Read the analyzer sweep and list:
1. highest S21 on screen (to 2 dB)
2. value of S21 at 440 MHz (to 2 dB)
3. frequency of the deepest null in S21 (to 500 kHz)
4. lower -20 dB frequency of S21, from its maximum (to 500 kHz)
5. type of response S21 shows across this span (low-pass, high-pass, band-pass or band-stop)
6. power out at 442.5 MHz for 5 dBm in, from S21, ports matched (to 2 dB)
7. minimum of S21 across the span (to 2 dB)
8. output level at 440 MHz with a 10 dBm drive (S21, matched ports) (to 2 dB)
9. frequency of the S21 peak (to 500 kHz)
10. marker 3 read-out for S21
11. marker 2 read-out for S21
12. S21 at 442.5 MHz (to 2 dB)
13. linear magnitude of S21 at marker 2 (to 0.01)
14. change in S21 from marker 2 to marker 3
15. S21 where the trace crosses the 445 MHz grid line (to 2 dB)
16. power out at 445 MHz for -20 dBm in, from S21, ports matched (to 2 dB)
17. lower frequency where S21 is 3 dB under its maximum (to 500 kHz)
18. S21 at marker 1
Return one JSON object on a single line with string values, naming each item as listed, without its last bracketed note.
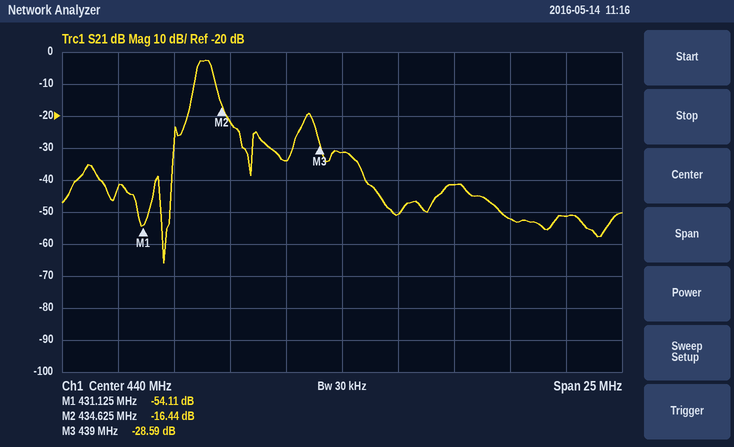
{"highest S21 on screen": "-2 dB", "value of S21 at 440 MHz": "-32 dB", "frequency of the deepest null in S21": "432.0 MHz", "lower -20 dB frequency of S21, from its maximum": "433.0 MHz", "type of response S21 shows across this span": "band-pass", "power out at 442.5 MHz for 5 dBm in, from S21, ports matched": "-46 dBm", "minimum of S21 across the span": "-66 dB", "output level at 440 MHz with a 10 dBm drive (S21, matched ports)": "-22 dBm", "frequency of the S21 peak": "434.0 MHz", "marker 3 read-out for S21": "-28.59 dB", "marker 2 read-out for S21": "-16.44 dB", "S21 at 442.5 MHz": "-50 dB", "linear magnitude of S21 at marker 2": "0.15", "change in S21 from marker 2 to marker 3": "-12.15 dB", "S21 where the trace crosses the 445 MHz grid line": "-42 dB", "power out at 445 MHz for -20 dBm in, from S21, ports matched": "-62 dBm", "lower frequency where S21 is 3 dB under its maximum": "433.5 MHz", "S21 at marker 1": "-54.11 dB"}
